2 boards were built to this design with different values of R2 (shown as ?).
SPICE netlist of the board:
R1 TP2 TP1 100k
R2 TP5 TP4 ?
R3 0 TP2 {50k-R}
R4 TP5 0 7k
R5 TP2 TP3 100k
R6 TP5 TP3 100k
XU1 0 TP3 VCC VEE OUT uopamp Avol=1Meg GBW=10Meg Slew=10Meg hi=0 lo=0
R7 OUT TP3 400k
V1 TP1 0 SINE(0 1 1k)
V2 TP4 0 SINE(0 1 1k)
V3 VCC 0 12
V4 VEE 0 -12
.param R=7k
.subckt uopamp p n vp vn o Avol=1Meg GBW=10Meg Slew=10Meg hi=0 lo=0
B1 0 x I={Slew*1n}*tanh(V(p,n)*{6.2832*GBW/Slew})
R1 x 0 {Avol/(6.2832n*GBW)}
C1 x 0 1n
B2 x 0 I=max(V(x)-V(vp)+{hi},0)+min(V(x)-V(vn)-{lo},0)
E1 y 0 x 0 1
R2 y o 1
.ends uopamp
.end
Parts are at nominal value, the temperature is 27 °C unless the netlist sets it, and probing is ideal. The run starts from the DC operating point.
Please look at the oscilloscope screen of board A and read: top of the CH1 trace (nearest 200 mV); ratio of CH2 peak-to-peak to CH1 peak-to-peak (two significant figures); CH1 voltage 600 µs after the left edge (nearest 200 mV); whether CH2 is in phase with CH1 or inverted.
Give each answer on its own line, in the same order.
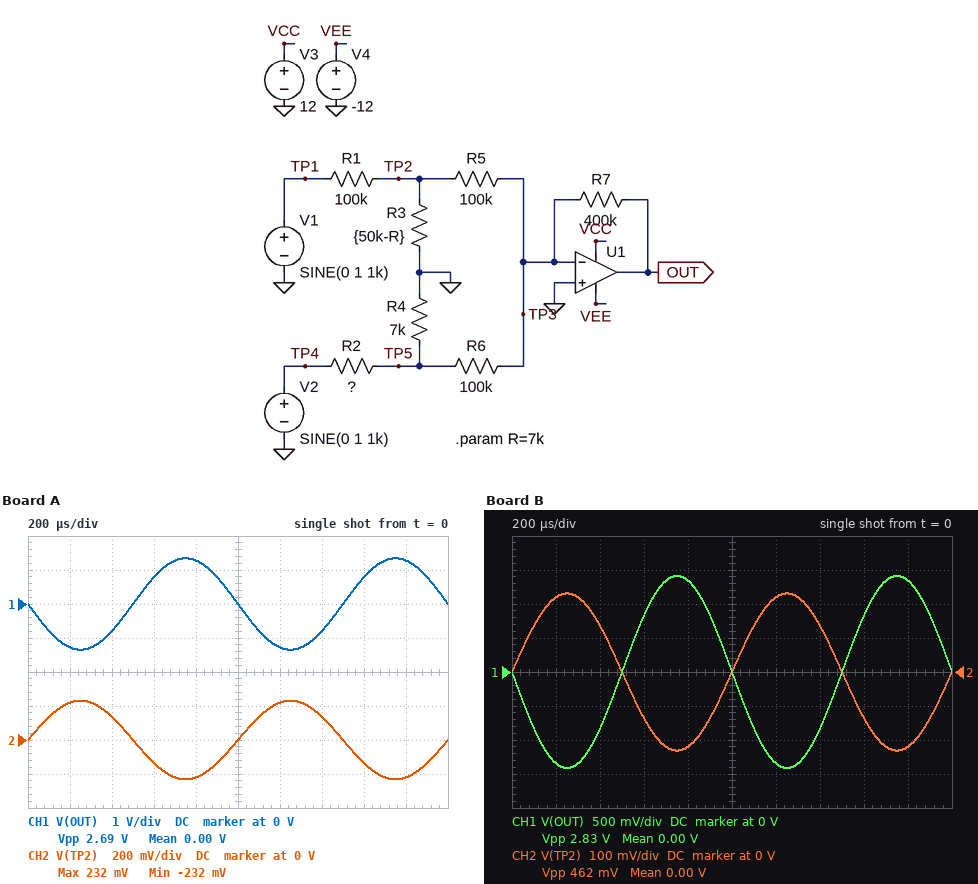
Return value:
1.4 V
0.17
800 mV
inverted
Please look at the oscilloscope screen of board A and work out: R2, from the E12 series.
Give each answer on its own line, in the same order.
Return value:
56 kΩ
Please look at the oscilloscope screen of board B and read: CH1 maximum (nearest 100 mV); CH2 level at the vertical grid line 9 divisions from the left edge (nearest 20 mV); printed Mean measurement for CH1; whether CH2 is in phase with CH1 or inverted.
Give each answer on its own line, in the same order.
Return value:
1.4 V
-220 mV
0.00 V
inverted
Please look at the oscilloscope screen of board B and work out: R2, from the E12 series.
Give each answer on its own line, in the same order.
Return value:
47 kΩ
